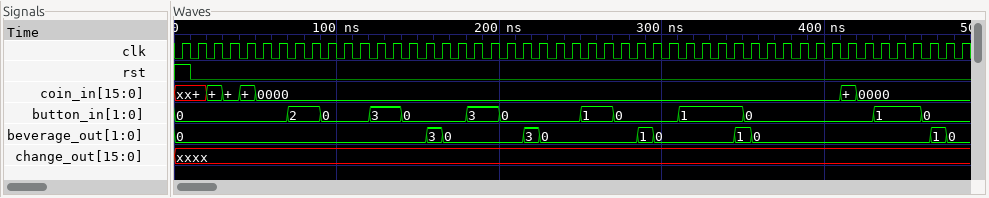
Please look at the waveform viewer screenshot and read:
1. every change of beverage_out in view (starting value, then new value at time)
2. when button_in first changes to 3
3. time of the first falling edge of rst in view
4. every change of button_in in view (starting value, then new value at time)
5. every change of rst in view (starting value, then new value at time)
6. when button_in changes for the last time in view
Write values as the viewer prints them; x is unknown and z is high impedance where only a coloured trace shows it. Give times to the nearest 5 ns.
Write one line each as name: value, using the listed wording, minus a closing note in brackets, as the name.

every change of beverage_out in view: 0, 3 at 155 ns, 0 at 165 ns, 3 at 215 ns, 0 at 225 ns, 1 at 285 ns, 0 at 295 ns, 1 at 345 ns, 0 at 355 ns, 1 at 465 ns, 0 at 475 ns
when button_in first changes to 3: 120 ns
time of the first falling edge of rst in view: 10 ns
every change of button_in in view: 0, 2 at 70 ns, 0 at 90 ns, 3 at 120 ns, 0 at 140 ns, 3 at 180 ns, 0 at 200 ns, 1 at 250 ns, 0 at 270 ns, 1 at 310 ns, 0 at 350 ns, 1 at 430 ns, 0 at 460 ns
every change of rst in view: 1, 0 at 10 ns
when button_in changes for the last time in view: 460 ns
